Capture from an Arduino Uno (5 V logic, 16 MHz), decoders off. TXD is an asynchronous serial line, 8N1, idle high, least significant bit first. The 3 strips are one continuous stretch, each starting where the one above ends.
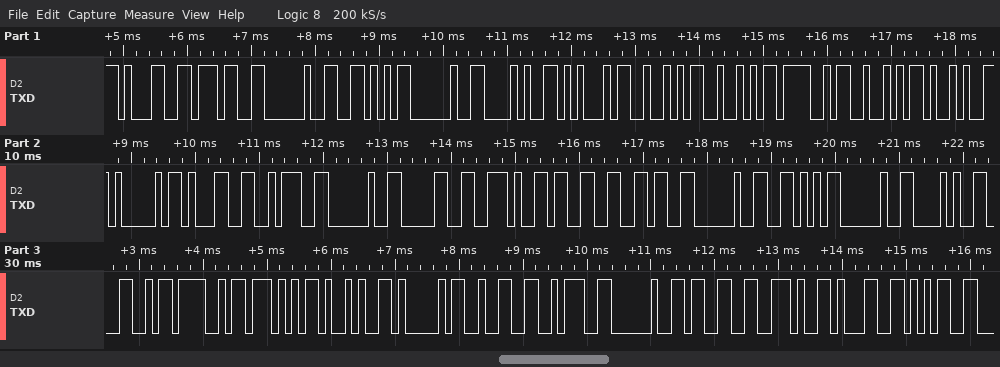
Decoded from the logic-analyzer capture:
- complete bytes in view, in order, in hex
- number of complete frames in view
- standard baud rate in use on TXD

31 37 20 56 20 28 45 52 52 4F 52 29 41 31 3A 20 30 2E 33 36 20 56 20 28 4C 4F 57 29 41 32 3A 20 33 2E 31 35
36
9600 baud
